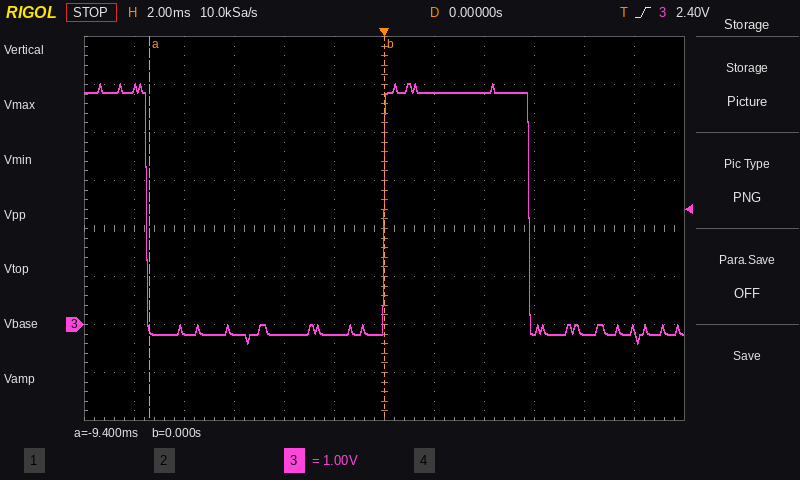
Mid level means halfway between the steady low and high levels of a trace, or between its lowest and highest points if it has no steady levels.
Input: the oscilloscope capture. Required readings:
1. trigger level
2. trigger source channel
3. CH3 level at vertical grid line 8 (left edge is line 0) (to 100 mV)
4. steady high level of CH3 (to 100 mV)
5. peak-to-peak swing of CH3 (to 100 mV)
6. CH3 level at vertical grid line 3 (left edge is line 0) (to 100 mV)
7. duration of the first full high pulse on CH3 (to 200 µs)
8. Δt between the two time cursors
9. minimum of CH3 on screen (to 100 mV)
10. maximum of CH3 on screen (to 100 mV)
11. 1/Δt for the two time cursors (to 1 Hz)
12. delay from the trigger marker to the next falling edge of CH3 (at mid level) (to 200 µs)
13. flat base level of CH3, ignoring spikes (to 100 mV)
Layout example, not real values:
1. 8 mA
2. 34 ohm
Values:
1. 2.40 V
2. CH3
3. 4.8 V
4. 4.8 V
5. 5.4 V
6. -200 mV
7. 5.8 ms
8. 9.4 ms
9. -400 mV
10. 5.0 V
11. 106 Hz
12. 5.8 ms
13. -200 mV
